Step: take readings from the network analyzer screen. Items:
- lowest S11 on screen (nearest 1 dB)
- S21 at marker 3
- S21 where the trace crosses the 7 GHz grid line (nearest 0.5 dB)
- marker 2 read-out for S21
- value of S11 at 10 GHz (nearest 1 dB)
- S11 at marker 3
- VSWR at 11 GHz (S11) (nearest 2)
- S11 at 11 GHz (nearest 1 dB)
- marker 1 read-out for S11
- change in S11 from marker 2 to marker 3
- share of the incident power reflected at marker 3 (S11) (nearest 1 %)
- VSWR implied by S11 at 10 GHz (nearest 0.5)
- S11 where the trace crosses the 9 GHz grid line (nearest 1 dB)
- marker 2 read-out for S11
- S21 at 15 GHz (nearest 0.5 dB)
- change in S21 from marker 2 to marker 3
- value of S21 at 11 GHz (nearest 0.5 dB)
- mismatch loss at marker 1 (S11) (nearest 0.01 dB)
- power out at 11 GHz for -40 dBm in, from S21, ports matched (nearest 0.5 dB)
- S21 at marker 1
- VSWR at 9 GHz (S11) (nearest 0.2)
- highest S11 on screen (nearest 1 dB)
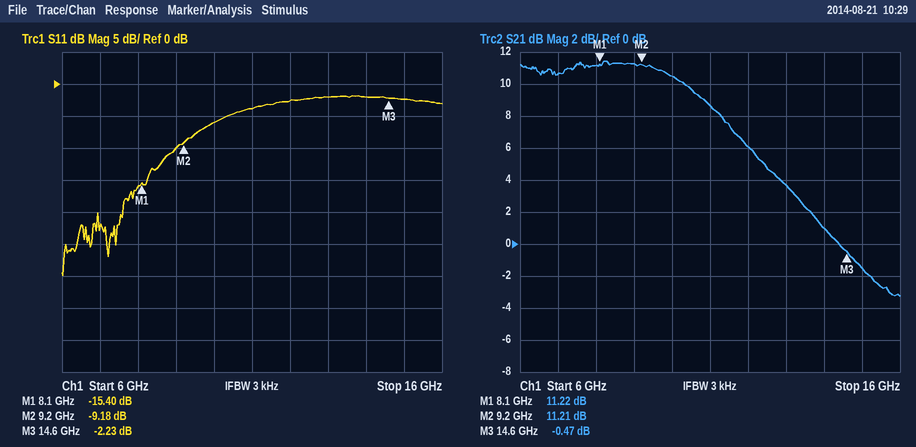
-30 dB
-0.47 dB
10.5 dB
11.21 dB
-6 dB
-2.23 dB
4
-4 dB
-15.40 dB
6.95 dB
60 %
3.0
-10 dB
-9.18 dB
-1.5 dB
-11.68 dB
8.5 dB
0.13 dB
-31.5 dBm
11.22 dB
2.0
-2 dB
